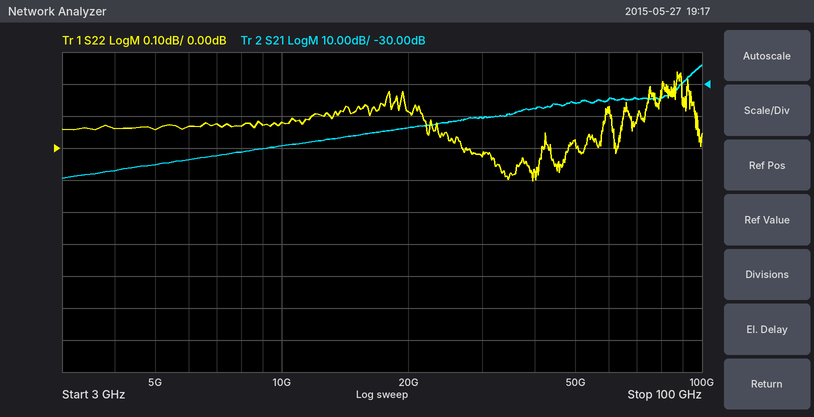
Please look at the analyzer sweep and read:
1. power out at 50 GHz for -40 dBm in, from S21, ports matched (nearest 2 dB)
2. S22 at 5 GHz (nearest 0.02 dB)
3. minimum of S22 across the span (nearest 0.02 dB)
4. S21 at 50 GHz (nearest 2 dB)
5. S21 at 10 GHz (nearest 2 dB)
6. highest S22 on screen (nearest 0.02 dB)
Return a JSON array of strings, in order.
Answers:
["-76 dBm", "0.06 dB", "-0.10 dB", "-36 dB", "-50 dB", "0.24 dB"]
